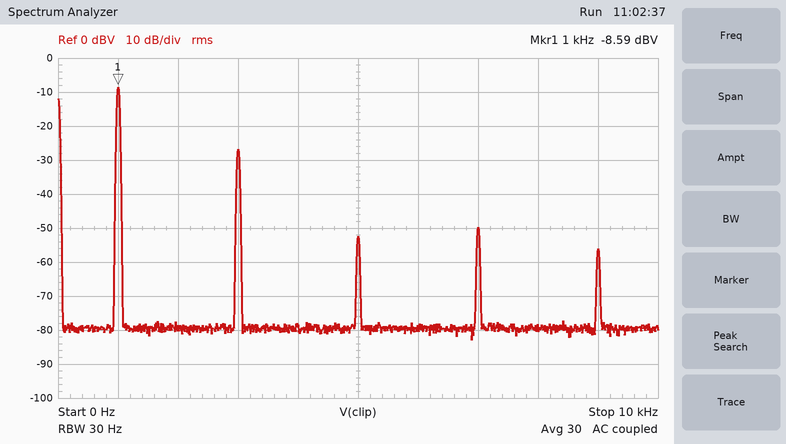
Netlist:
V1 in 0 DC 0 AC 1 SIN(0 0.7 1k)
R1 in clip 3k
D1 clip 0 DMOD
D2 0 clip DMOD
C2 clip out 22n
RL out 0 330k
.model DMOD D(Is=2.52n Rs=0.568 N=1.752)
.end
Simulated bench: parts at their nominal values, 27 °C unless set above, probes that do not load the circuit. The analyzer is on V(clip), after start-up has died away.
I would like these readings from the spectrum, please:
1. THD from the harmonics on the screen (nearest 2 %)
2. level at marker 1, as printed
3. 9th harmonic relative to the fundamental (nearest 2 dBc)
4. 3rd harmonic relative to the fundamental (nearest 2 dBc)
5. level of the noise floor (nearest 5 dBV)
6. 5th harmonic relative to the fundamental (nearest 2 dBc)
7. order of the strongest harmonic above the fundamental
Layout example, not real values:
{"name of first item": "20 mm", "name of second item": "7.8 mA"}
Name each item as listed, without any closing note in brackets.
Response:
{"THD from the harmonics on the screen": "12 %", "level at marker 1, as printed": "-8.59 dBV", "9th harmonic relative to the fundamental": "-48 dBc", "3rd harmonic relative to the fundamental": "-18 dBc", "level of the noise floor": "-80 dBV", "5th harmonic relative to the fundamental": "-44 dBc", "order of the strongest harmonic above the fundamental": "3"}
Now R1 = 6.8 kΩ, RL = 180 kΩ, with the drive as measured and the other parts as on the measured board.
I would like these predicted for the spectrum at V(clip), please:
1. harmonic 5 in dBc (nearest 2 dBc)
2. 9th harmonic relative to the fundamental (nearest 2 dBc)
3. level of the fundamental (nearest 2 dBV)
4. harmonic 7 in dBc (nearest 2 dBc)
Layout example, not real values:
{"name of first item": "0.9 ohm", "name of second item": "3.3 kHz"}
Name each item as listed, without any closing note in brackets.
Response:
{"harmonic 5 in dBc": "-38 dBc", "9th harmonic relative to the fundamental": "-46 dBc", "level of the fundamental": "-10 dBV", "harmonic 7 in dBc": "-44 dBc"}
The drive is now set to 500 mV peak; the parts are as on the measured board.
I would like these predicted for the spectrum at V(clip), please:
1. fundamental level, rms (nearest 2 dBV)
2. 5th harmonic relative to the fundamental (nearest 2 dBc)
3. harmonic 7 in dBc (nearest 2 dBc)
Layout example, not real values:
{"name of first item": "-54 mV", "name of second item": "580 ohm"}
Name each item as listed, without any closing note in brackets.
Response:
{"fundamental level, rms": "-10 dBV", "5th harmonic relative to the fundamental": "-40 dBc", "harmonic 7 in dBc": "-52 dBc"}
